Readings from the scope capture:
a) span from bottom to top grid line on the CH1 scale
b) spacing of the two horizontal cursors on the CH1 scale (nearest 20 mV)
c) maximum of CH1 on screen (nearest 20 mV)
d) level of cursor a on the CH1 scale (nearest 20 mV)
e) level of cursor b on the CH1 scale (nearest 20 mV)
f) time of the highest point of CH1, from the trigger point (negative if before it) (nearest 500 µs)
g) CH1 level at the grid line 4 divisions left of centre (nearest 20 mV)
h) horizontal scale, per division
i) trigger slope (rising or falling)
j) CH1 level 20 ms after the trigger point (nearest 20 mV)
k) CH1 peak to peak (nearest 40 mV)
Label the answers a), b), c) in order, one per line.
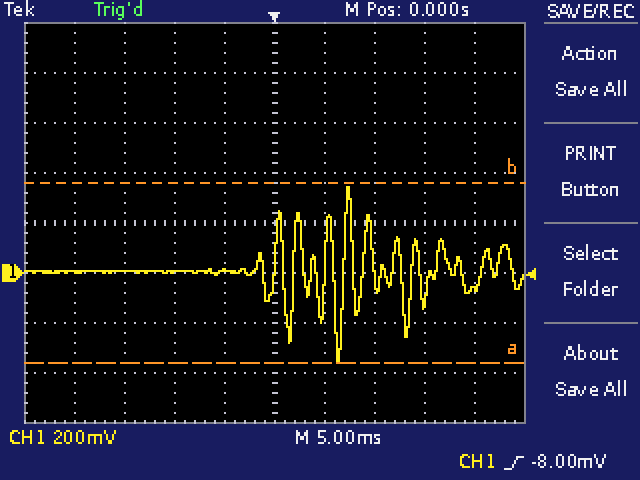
a) 1.6 V
b) 720 mV
c) 340 mV
d) -360 mV
e) 360 mV
f) +7.5 ms
g) 0 mV
h) 5 ms
i) rising
j) -60 mV
k) 680 mV
